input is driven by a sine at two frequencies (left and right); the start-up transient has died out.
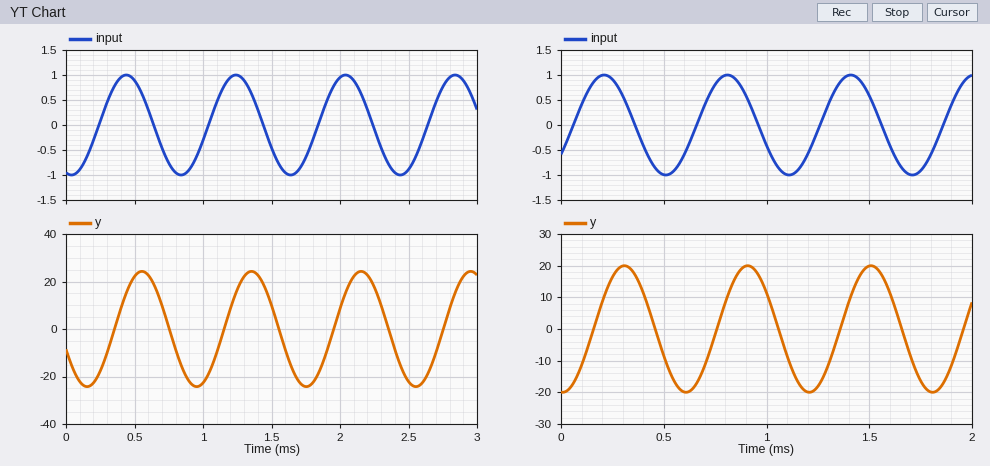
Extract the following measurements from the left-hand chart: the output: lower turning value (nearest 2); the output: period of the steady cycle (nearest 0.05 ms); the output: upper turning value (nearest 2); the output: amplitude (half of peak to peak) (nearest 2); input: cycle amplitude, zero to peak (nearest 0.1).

-24
0.80 ms
24
24
1.0
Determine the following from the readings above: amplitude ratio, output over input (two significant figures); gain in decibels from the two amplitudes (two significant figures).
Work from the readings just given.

24
28 dB
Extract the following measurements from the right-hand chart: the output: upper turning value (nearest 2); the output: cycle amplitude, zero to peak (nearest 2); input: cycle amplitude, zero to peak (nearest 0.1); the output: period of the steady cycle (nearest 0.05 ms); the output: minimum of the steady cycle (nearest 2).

20
20
1.0
0.60 ms
-20
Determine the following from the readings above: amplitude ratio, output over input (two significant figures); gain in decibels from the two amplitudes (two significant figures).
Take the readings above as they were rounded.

20
26 dB
